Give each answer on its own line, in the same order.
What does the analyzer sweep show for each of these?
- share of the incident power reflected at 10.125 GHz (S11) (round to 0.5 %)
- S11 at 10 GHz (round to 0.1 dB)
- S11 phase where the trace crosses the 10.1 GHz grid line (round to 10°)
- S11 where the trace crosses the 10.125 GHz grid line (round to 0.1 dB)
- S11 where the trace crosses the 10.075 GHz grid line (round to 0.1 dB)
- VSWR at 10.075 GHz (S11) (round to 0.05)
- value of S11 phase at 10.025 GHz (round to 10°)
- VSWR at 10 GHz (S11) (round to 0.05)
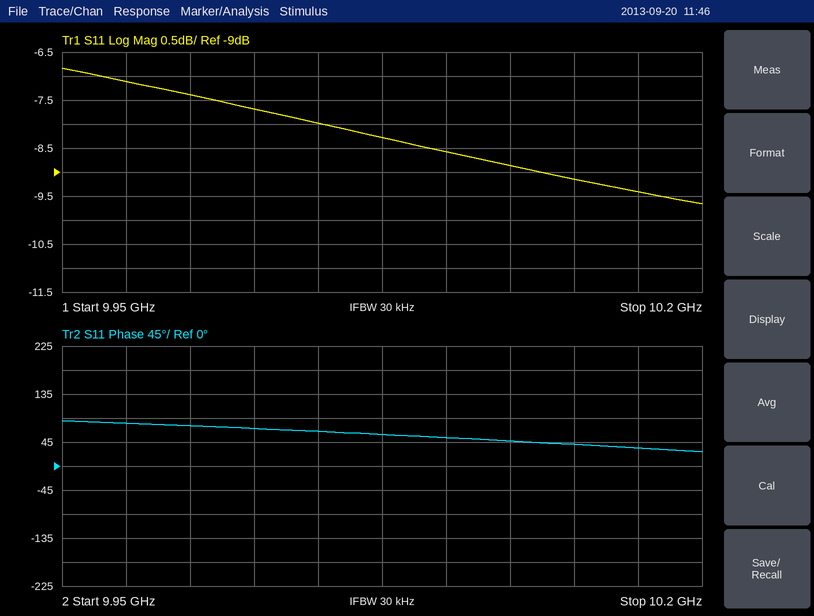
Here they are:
13.0 %
-7.4 dB
50°
-8.9 dB
-8.3 dB
2.25
70°
2.50
